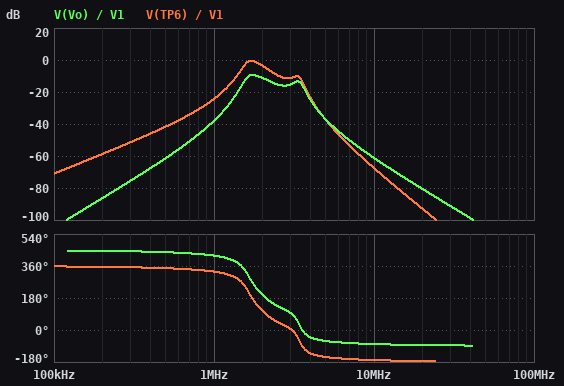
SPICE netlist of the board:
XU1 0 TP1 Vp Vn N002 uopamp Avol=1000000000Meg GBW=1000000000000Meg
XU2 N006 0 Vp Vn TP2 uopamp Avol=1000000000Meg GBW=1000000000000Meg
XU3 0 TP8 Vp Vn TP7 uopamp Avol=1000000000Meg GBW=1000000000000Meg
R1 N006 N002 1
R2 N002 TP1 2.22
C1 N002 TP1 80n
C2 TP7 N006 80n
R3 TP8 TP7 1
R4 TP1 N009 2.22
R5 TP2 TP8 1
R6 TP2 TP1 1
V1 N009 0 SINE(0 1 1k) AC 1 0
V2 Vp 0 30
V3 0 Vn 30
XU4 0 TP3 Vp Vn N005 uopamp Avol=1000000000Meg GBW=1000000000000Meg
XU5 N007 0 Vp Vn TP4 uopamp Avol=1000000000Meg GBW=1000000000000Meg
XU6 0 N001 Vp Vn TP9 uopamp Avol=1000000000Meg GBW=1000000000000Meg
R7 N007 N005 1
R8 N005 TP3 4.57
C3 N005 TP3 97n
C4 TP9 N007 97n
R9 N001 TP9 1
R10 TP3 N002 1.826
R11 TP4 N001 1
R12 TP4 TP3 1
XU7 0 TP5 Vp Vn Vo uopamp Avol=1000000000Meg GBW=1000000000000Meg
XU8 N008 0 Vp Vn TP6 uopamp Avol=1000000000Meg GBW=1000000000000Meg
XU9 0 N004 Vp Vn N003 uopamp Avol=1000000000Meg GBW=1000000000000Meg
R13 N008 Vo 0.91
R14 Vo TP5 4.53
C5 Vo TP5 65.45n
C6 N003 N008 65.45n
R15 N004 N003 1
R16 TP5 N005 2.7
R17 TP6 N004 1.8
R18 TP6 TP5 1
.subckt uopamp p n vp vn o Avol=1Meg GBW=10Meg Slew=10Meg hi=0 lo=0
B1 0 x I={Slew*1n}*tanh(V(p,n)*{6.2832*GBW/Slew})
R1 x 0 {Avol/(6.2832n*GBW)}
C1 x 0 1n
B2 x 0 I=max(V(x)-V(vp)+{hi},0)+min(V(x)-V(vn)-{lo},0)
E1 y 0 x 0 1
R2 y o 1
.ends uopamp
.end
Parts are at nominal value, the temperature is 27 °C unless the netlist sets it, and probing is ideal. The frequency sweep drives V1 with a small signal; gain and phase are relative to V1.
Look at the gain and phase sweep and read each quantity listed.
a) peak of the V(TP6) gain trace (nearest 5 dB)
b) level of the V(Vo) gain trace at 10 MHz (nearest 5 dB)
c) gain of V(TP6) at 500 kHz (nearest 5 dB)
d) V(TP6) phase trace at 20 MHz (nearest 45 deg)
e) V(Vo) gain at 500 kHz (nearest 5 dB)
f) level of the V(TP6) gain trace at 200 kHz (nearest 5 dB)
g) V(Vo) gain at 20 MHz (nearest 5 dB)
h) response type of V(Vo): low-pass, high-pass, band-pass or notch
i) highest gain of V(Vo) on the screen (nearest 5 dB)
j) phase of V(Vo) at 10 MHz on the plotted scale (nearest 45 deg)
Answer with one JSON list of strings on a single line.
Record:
["0 dB", "-60 dB", "-40 dB", "-180 deg", "-60 dB", "-60 dB", "-80 dB", "band-pass", "-10 dB", "-90 deg"]
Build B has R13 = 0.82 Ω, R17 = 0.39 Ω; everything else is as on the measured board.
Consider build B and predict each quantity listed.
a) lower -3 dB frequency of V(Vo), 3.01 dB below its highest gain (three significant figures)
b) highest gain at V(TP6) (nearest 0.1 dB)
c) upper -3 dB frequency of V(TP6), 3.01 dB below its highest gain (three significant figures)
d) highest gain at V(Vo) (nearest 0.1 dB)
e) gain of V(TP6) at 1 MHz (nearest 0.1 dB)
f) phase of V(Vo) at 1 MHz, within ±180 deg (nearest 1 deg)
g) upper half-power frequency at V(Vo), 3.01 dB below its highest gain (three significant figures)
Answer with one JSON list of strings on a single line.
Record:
["1.56 MHz", "7.1 dB", "1.82 MHz", "10.3 dB", "-21.6 dB", "45 deg", "1.85 MHz"]
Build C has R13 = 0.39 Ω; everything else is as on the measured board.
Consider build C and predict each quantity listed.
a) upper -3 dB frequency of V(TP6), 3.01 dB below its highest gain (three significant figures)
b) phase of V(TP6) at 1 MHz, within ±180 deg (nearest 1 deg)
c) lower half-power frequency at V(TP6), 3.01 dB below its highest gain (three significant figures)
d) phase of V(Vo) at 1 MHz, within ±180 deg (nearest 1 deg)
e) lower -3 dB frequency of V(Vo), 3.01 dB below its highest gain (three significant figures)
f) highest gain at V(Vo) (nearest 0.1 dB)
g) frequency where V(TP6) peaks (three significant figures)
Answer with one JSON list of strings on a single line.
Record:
["1.95 MHz", "-30 deg", "1.54 MHz", "60 deg", "1.56 MHz", "-18.2 dB", "1.69 MHz"]
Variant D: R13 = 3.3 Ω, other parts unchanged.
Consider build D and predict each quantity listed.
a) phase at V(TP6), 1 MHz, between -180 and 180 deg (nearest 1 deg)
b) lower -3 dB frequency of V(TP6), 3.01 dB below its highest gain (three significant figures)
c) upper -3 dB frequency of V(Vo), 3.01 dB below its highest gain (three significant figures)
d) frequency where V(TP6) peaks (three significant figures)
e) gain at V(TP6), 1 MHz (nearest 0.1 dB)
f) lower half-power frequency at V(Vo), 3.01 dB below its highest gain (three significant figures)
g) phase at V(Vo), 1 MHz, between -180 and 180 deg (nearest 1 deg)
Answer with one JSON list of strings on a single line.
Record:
["-42 deg", "1.57 MHz", "1.91 MHz", "1.71 MHz", "-22.1 dB", "1.59 MHz", "48 deg"]
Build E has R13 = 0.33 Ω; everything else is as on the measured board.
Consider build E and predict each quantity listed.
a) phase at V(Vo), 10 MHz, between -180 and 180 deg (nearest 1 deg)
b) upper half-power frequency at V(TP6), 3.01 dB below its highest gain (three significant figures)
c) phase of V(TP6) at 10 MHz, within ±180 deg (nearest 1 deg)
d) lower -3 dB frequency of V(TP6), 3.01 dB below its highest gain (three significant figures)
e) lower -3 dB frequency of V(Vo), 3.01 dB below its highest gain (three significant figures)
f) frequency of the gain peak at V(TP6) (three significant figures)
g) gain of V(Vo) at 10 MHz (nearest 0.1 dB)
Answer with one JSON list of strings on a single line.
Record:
["-78 deg", "1.95 MHz", "-168 deg", "1.54 MHz", "1.56 MHz", "1.69 MHz", "-58.9 dB"]
